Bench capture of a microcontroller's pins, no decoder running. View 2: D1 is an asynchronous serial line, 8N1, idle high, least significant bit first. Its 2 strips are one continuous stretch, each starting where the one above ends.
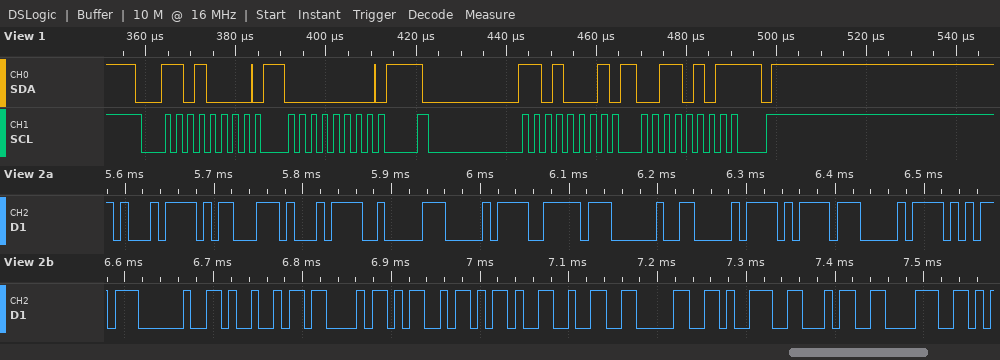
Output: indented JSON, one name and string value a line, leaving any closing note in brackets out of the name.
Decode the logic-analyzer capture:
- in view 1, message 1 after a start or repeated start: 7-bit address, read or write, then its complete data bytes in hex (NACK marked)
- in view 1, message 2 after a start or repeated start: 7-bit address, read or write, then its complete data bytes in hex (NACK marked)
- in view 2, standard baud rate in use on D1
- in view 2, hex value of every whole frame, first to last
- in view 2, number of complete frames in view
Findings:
{
  "in view 1, message 1 after a start or repeated start: 7-bit address, read or write, then its complete data bytes in hex": "0x68 write: 00",
  "in view 1, message 2 after a start or repeated start: 7-bit address, read or write, then its complete data bytes in hex": "0x68 read: 35 NACK",
  "in view 2, standard baud rate in use on D1": "115200 baud",
  "in view 2, hex value of every whole frame, first to last": "D1 8D D1 82 D0 BE 20 D0 BD D0 B5 20 49 43 4D 2D 32 30 39 34 38",
  "in view 2, number of complete frames in view": "21"
}
